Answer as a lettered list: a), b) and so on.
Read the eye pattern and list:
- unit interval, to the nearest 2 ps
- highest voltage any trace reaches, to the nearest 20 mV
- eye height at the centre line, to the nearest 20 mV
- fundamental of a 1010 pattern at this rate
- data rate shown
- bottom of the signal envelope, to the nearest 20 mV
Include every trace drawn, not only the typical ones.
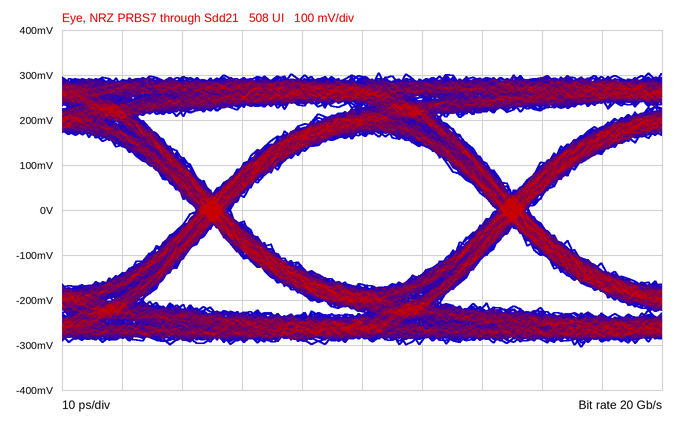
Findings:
a) 50 ps
b) 300 mV
c) 340 mV
d) 10 GHz
e) 20 Gb/s
f) -300 mV
